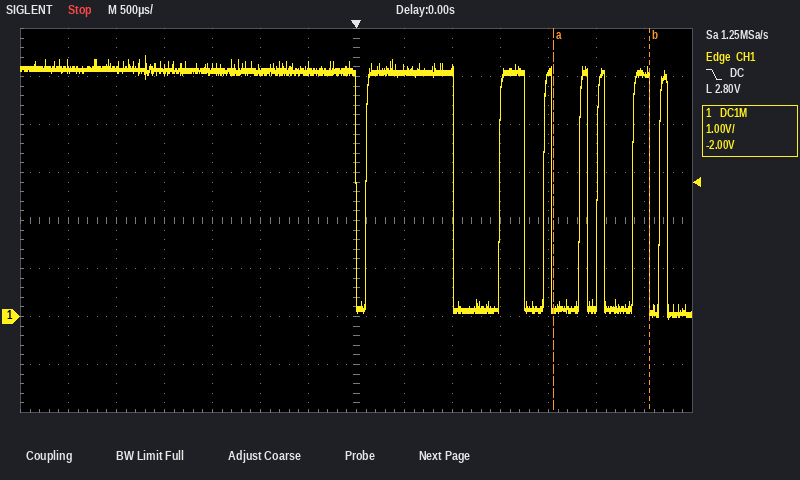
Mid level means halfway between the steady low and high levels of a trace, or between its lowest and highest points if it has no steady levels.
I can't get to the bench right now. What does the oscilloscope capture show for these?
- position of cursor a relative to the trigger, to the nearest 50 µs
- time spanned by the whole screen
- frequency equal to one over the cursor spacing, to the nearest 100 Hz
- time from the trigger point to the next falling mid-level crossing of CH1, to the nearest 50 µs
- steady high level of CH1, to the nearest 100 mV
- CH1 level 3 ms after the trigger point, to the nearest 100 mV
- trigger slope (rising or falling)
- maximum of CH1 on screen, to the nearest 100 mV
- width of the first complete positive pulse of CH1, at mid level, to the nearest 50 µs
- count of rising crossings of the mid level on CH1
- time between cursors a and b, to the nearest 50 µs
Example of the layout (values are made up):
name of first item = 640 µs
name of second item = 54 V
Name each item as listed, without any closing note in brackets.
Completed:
position of cursor a relative to the trigger, to the nearest 50 µs = +2.05 ms
time spanned by the whole screen = 7 ms
frequency equal to one over the cursor spacing, to the nearest 100 Hz = 1.0 kHz
time from the trigger point to the next falling mid-level crossing of CH1, to the nearest 50 µs = 1.00 ms
steady high level of CH1, to the nearest 100 mV = 5.1 V
CH1 level 3 ms after the trigger point, to the nearest 100 mV = 5.1 V
trigger slope = falling
maximum of CH1 on screen, to the nearest 100 mV = 5.4 V
width of the first complete positive pulse of CH1, at mid level, to the nearest 50 µs = 900 µs
count of rising crossings of the mid level on CH1 = 7
time between cursors a and b, to the nearest 50 µs = 1.00 ms
